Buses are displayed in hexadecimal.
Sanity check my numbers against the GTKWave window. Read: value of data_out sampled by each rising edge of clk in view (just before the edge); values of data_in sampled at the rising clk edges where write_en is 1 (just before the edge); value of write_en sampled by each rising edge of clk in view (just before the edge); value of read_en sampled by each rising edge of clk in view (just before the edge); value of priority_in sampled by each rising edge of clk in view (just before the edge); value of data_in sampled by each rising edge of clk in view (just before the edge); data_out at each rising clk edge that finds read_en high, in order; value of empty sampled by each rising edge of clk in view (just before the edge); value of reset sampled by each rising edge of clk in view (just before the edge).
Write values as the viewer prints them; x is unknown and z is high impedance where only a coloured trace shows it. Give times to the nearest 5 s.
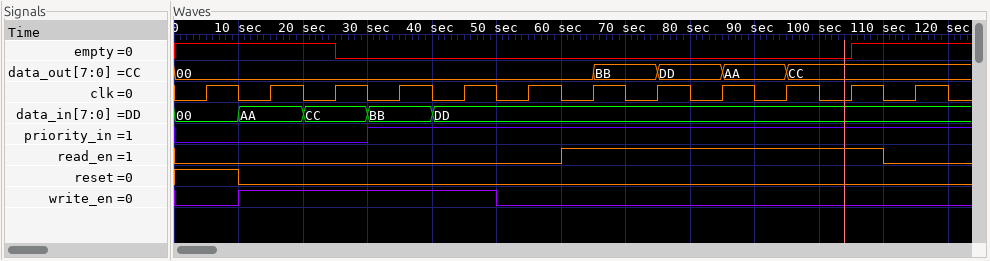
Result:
00, 00, 00, 00, 00, 00, 00, BB, DD, AA, CC, CC
AA, CC, BB, DD
0 1 1 1 1 0 0 0 0 0 0 0
0 0 0 0 0 0 1 1 1 1 1 0
0 0 0 1 1 1 1 1 1 1 1 1
00, AA, CC, BB, DD, DD, DD, DD, DD, DD, DD, DD
00, BB, DD, AA, CC
1 1 1 0 0 0 0 0 0 0 0 1
1 0 0 0 0 0 0 0 0 0 0 0
